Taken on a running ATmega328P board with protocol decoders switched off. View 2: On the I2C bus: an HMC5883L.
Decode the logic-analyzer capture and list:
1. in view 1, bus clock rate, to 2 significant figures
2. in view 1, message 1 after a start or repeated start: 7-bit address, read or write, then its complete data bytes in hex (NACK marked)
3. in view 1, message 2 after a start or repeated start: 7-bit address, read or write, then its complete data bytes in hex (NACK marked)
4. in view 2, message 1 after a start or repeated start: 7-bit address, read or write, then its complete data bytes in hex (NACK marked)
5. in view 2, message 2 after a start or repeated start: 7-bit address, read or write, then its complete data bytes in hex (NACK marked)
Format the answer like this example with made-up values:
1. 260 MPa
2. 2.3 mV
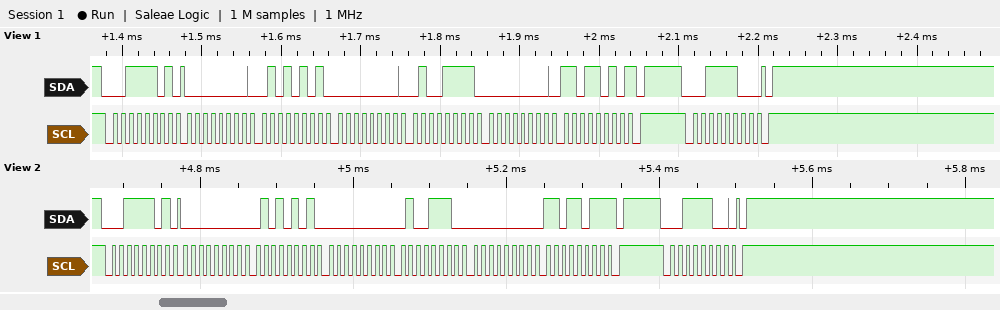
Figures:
1. 100 kHz
2. 0x1E read: 00 55 00 4F 00 DA NACK
3. 0x1E write
4. 0x1E read: 00 55 00 4E 00 DB NACK
5. 0x1E write
